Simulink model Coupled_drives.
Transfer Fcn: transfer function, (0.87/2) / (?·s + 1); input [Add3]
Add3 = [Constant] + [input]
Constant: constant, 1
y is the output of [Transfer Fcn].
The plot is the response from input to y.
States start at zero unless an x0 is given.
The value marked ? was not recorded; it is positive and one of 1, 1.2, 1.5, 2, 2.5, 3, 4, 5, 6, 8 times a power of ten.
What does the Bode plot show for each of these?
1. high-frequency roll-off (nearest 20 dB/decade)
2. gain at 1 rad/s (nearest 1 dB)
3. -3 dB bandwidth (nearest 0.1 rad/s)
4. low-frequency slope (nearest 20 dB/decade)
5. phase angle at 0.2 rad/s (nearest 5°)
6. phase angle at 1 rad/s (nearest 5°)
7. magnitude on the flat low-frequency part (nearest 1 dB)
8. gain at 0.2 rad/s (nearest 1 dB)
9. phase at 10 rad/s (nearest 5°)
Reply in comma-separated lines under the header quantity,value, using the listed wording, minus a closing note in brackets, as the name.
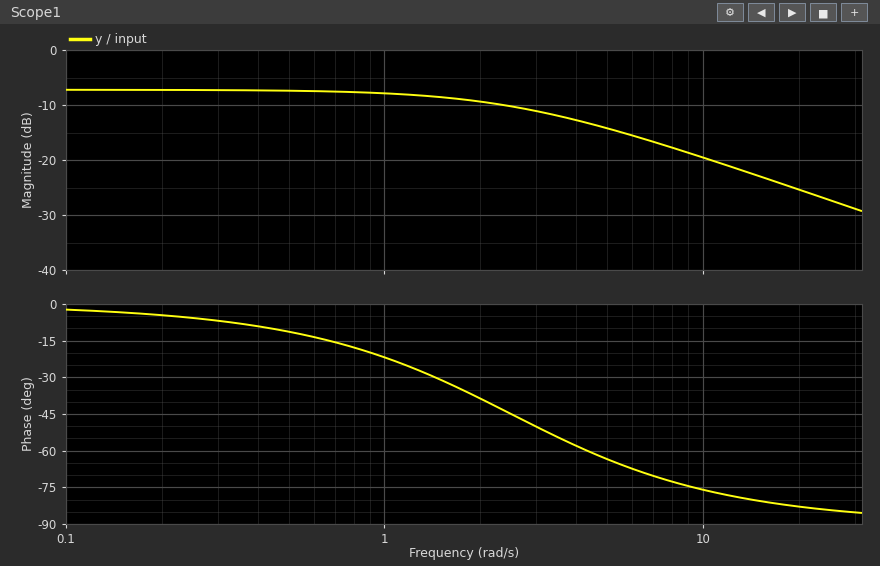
quantity,value
high-frequency roll-off,-20 dB/decade
gain at 1 rad/s,-8 dB
-3 dB bandwidth,2.5 rad/s
low-frequency slope,0 dB/decade
phase angle at 0.2 rad/s,-5°
phase angle at 1 rad/s,-20°
magnitude on the flat low-frequency part,-7 dB
gain at 0.2 rad/s,-7 dB
phase at 10 rad/s,-75°
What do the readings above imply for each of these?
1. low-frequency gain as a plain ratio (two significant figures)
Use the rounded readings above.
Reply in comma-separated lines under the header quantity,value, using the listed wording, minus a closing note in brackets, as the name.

quantity,value
low-frequency gain as a plain ratio,0.45
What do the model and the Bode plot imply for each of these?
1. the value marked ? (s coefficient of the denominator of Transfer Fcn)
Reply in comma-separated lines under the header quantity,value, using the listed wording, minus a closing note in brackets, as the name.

quantity,value
the value marked ?,0.4
